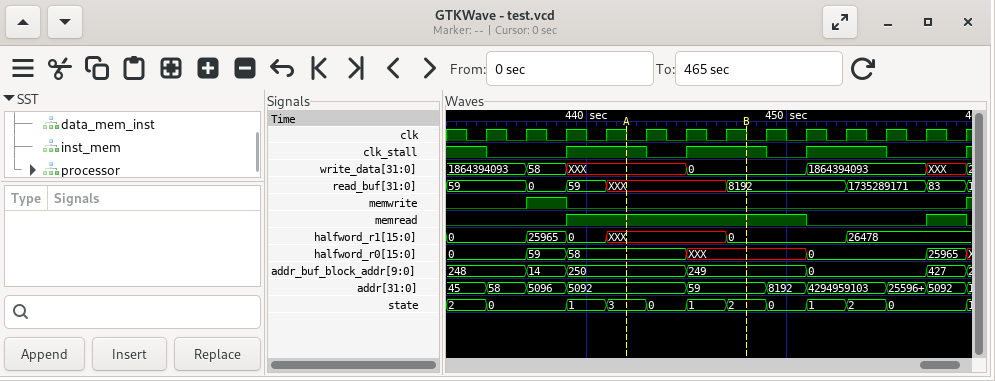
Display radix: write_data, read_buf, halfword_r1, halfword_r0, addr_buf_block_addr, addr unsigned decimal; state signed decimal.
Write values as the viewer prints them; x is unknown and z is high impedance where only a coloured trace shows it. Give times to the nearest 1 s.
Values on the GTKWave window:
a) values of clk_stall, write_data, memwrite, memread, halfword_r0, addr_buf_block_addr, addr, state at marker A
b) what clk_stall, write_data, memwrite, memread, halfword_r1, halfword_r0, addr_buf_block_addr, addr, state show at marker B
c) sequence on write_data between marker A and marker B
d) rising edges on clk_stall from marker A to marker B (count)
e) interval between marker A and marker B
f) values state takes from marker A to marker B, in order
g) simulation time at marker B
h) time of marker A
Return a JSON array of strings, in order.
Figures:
["clk_stall=1, write_data=XXX, memwrite=0, memread=1, halfword_r0=58, addr_buf_block_addr=250, addr=5092, state=3", "clk_stall=1, write_data=0, memwrite=0, memread=1, halfword_r1=0, halfword_r0=XXX, addr_buf_block_addr=249, addr=59, state=2", "XXX, 0", "1", "6 s", "3, 0, 1, 2", "448 s", "442 s"]
